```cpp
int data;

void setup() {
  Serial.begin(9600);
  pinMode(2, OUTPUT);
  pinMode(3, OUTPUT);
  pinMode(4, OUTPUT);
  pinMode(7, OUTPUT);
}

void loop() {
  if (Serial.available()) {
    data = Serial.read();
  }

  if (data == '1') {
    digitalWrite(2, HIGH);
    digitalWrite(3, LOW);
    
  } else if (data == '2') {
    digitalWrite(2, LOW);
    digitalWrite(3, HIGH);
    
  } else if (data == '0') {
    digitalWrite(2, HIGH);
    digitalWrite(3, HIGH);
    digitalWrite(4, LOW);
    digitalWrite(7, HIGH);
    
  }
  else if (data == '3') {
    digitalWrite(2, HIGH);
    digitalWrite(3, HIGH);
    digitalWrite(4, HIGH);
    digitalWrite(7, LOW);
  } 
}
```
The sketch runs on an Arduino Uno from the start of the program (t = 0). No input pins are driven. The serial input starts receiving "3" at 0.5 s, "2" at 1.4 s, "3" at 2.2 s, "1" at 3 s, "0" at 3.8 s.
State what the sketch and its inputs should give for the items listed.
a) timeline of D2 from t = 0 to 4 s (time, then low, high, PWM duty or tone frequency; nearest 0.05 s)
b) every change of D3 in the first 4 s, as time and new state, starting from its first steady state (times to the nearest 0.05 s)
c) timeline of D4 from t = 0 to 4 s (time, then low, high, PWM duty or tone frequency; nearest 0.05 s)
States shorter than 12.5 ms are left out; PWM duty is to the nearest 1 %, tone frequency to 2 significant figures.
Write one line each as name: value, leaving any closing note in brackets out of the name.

timeline of D2 from t = 0 to 4 s: 0 s low; 0.5 s high; 1.4 s low; 2.2 s high
every change of D3 in the first 4 s, as time and new state, starting from its first steady state: 0 s low; 0.5 s high; 3 s low; 3.8 s high
timeline of D4 from t = 0 to 4 s: 0 s low; 0.5 s high; 3.8 s low
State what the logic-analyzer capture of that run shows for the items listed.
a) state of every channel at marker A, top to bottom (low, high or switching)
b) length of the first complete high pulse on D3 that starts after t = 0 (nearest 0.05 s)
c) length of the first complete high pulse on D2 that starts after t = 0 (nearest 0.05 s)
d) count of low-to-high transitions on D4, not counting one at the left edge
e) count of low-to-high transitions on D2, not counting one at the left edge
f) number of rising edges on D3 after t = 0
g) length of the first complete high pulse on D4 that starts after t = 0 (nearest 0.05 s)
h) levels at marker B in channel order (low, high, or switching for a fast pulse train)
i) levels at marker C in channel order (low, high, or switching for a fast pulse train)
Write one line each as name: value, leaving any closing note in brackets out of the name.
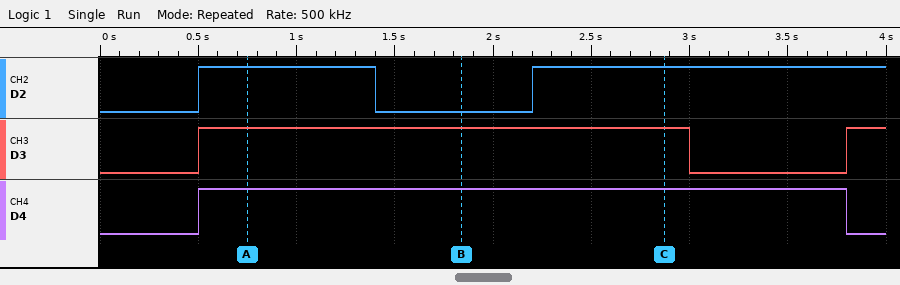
state of every channel at marker A, top to bottom: D2 high, D3 high, D4 high
length of the first complete high pulse on D3 that starts after t = 0: 2.50 s
length of the first complete high pulse on D2 that starts after t = 0: 0.90 s
count of low-to-high transitions on D4, not counting one at the left edge: 1
count of low-to-high transitions on D2, not counting one at the left edge: 2
number of rising edges on D3 after t = 0: 2
length of the first complete high pulse on D4 that starts after t = 0: 3.30 s
levels at marker B in channel order: D2 low, D3 high, D4 high
levels at marker C in channel order: D2 high, D3 high, D4 high
